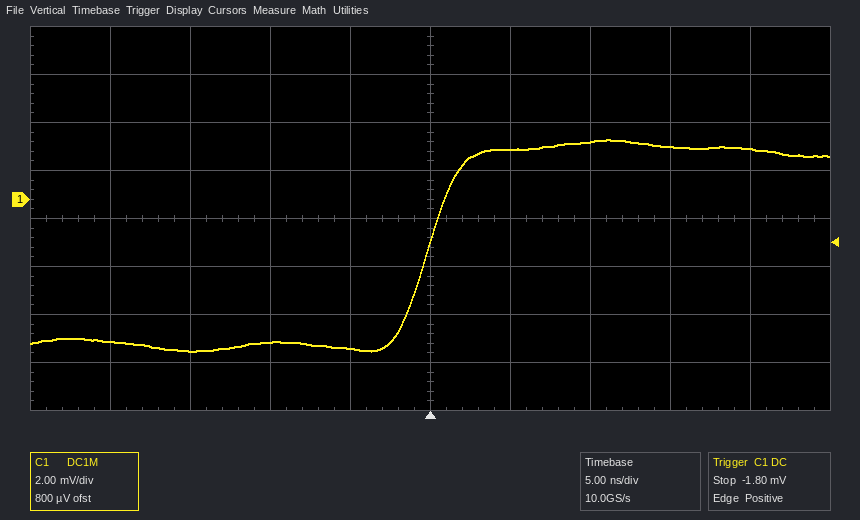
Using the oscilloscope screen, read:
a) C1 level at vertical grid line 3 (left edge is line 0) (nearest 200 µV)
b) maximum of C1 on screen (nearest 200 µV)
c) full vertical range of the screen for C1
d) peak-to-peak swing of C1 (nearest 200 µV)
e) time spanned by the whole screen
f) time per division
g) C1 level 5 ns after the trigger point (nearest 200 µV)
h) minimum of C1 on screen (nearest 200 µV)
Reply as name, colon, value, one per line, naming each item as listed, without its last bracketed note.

C1 level at vertical grid line 3 (left edge is line 0): -6.0 mV
maximum of C1 on screen: 2.4 mV
full vertical range of the screen for C1: 16 mV
peak-to-peak swing of C1: 8.8 mV
time spanned by the whole screen: 50 ns
time per division: 5 ns
C1 level 5 ns after the trigger point: 2.0 mV
minimum of C1 on screen: -6.4 mV
